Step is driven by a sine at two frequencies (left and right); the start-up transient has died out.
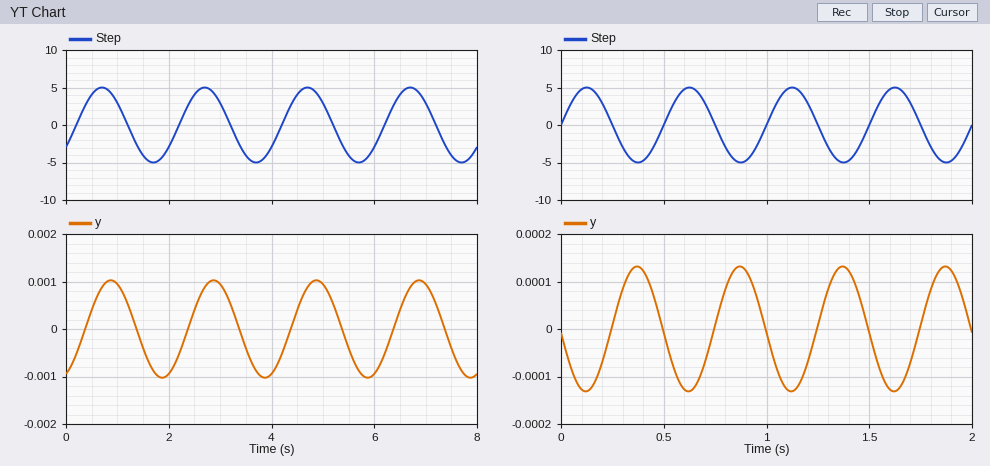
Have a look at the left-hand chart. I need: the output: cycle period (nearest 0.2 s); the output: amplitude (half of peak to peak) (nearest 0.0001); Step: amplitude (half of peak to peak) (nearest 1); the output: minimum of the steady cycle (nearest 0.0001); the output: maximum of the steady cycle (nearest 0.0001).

2.0 s
0.0010
5
-0.0010
0.0010
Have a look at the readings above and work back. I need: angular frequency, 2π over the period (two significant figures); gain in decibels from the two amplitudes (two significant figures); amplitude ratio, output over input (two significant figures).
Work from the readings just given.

3.1 rad/s
-74 dB
0.00020
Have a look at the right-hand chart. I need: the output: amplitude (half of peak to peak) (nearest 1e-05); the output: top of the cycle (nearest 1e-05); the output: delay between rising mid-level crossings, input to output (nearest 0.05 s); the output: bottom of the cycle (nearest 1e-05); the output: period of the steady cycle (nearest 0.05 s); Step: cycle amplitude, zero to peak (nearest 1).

0.00013
0.00013
0.25 s
-0.00013
0.50 s
5
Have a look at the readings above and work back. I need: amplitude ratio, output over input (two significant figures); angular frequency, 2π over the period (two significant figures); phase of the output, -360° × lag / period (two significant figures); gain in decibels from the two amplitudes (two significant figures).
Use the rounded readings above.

0.000026
13 rad/s
-180°
-92 dB
